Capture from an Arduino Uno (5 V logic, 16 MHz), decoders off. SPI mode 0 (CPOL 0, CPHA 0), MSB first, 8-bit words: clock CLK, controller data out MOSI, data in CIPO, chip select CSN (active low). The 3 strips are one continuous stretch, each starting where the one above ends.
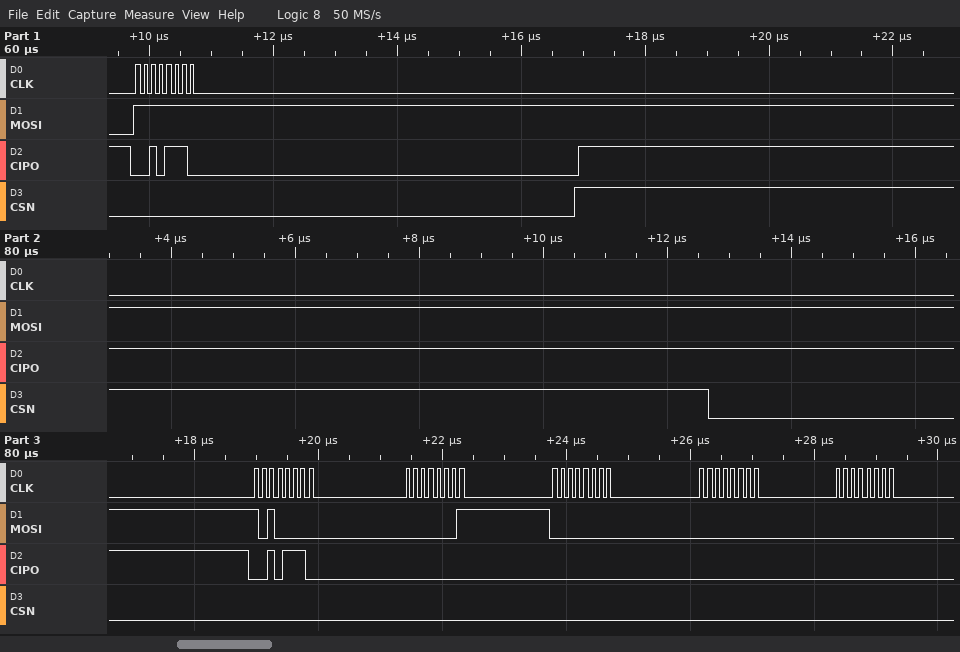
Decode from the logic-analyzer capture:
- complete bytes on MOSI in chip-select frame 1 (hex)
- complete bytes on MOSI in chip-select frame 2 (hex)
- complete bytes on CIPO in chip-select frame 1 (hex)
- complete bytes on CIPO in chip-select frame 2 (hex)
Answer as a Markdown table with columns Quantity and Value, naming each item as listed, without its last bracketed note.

| Quantity | Value |
|---|---|
| complete bytes on MOSI in chip-select frame 1 | FF |
| complete bytes on MOSI in chip-select frame 2 | A0 01 00 00 00 |
| complete bytes on CIPO in chip-select frame 1 | 2E |
| complete bytes on CIPO in chip-select frame 2 | 2E 00 00 00 00 |
